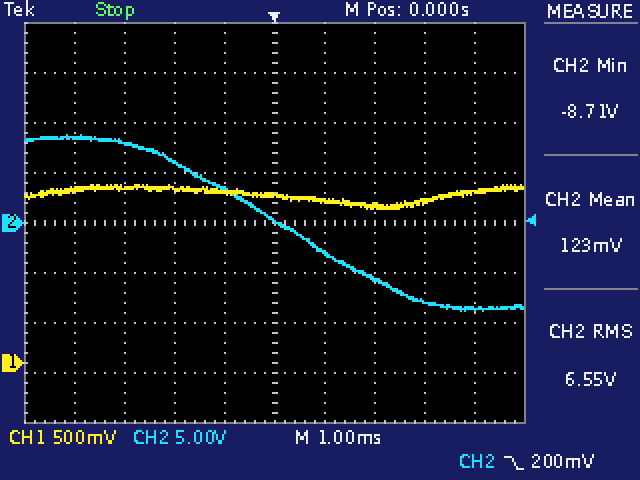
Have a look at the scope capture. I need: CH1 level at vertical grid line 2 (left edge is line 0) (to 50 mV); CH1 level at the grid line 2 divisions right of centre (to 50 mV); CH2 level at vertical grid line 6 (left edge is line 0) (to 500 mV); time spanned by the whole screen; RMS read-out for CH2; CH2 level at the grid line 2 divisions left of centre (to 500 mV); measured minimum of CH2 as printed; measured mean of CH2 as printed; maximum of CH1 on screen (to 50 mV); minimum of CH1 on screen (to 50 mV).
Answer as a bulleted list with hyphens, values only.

- 1.75 V
- 1.55 V
- -3.0 V
- 10 ms
- 6.55 V
- 6.0 V
- -8.71 V
- 123 mV
- 1.80 V
- 1.55 V
